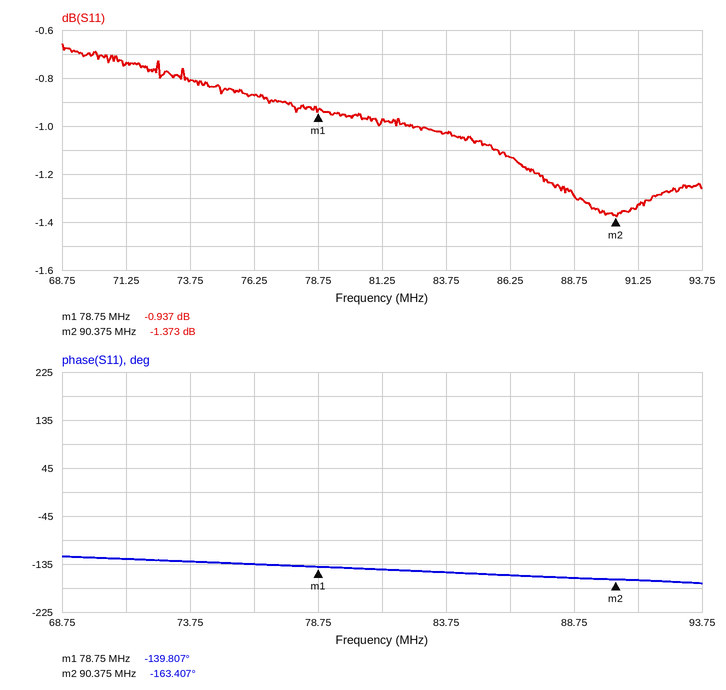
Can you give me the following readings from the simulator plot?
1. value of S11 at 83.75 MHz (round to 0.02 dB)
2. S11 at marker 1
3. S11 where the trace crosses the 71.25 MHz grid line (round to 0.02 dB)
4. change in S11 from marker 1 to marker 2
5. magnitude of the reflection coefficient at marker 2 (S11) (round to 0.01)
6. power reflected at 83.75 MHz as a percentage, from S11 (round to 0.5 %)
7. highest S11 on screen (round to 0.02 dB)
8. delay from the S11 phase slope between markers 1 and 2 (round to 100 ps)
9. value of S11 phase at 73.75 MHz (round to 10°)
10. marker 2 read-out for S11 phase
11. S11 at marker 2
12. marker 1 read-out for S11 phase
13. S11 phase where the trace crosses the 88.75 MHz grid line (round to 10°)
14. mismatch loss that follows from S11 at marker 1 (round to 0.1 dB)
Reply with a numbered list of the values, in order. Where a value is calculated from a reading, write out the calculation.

1. -1.02 dB
2. -0.937 dB
3. -0.74 dB
4. -1.373 − (-0.937) = -0.436 dB
5. 10^(-1.373/20) ≈ 0.85
6. 10^(-1.02/10) ≈ 79.1 %, so 79.0 % to the nearest 0.5 %
7. -0.66 dB
8. −(-163.407° − (-139.807°))/(360° × 11.625 MHz) ≈ 5.6 ns
9. -130°
10. -163.407°
11. -1.373 dB
12. -139.807°
13. -160°
14. −10 log10(1 − 10^(-0.937/10)) ≈ 7.1 dB
